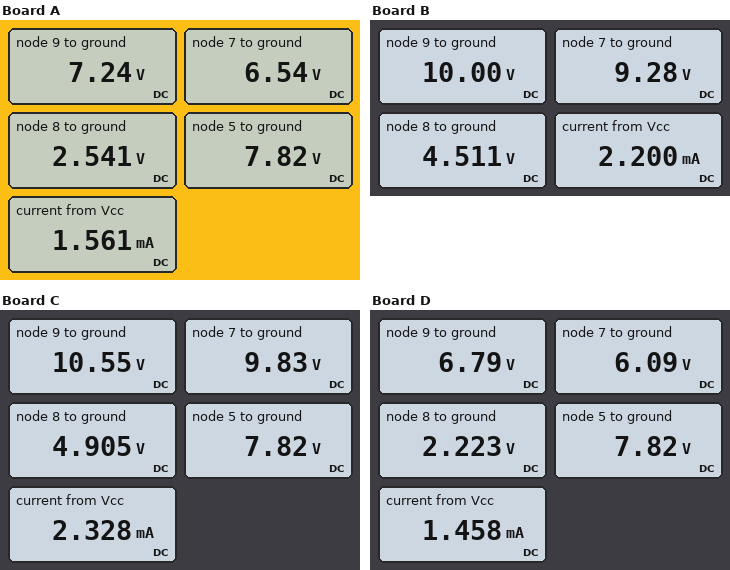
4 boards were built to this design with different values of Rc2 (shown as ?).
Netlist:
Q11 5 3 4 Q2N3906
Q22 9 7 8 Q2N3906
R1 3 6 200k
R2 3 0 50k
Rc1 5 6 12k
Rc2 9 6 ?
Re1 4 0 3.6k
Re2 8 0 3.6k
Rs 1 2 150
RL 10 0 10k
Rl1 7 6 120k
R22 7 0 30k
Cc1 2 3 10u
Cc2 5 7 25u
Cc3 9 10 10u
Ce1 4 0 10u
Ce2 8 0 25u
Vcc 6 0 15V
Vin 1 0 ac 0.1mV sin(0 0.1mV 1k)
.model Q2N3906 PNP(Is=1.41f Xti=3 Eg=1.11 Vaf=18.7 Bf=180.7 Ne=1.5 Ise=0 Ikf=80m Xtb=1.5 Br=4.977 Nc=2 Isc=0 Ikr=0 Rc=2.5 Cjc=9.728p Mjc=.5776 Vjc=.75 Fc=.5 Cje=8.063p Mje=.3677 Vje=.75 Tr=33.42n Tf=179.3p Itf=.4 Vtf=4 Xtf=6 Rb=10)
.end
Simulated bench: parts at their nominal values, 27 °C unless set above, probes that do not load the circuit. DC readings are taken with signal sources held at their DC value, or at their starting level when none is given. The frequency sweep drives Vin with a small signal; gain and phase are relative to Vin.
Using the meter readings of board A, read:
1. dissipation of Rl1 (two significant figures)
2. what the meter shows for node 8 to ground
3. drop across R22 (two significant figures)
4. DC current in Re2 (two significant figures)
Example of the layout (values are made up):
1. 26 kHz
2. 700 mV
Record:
1. 600 µW
2. 2.541 V
3. 6.5 V
4. 710 µA
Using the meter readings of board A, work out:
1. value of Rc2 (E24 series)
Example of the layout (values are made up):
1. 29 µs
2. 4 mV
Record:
1. 9.1 kΩ
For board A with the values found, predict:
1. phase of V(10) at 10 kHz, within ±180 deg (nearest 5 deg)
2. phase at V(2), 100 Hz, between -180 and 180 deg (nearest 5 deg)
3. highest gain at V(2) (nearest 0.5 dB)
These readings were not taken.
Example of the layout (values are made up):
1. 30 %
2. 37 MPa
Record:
1. 0 deg
2. 0 deg
3. 0 dB
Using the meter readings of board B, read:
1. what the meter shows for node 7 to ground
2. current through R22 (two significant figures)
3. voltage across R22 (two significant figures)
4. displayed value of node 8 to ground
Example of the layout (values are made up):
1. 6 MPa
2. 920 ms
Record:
1. 9.28 V
2. 310 µA
3. 9.3 V
4. 4.511 V
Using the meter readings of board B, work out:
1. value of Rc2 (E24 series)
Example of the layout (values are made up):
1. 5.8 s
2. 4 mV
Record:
1. 3.3 kΩ
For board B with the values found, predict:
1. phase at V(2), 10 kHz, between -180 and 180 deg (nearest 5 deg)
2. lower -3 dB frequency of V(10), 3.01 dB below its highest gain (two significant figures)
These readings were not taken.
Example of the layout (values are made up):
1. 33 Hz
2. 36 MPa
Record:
1. 0 deg
2. 2.3 Hz
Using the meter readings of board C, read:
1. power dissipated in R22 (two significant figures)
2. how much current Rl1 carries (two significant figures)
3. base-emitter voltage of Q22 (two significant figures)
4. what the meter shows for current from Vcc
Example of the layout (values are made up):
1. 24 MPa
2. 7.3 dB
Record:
1. 3.2 mW
2. 43 µA
3. 4.9 V
4. 2.328 mA
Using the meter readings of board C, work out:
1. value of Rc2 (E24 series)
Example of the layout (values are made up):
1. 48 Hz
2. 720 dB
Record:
1. 2.7 kΩ
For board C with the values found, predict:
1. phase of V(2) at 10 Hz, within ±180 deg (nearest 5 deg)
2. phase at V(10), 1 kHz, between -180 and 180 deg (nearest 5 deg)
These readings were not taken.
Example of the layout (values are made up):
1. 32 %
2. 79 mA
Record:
1. 0 deg
2. 0 deg
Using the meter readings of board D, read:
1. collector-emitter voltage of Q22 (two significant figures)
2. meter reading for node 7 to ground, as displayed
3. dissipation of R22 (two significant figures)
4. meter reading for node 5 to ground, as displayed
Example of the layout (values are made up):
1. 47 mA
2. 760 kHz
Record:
1. 4.6 V
2. 6.09 V
3. 1.2 mW
4. 7.82 V
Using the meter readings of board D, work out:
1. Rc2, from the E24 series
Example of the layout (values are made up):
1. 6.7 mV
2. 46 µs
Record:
1. 11 kΩ
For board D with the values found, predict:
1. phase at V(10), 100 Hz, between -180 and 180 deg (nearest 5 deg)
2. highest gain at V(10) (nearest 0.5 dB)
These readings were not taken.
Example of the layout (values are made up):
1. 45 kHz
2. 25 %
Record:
1. 0 deg
2. 0 dB
